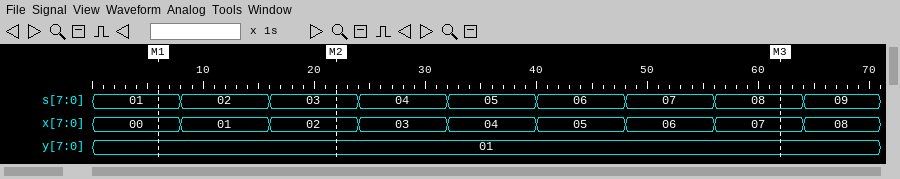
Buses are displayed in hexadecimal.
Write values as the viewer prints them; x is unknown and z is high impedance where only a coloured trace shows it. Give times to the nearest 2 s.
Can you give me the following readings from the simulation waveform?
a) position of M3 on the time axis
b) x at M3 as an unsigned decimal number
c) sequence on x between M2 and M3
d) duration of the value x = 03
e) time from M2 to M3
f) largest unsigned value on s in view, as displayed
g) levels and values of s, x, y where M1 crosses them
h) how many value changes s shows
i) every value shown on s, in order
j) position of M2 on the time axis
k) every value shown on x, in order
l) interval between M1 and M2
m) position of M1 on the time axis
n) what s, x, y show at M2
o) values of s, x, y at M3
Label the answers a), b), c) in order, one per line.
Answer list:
a) 62 s
b) 7
c) 02, 03, 04, 05, 06, 07
d) 8 s
e) 40 s
f) 09
g) s=01, x=00, y=01
h) 8
i) 01, 02, 03, 04, 05, 06, 07, 08, 09
j) 22 s
k) 00, 01, 02, 03, 04, 05, 06, 07, 08
l) 16 s
m) 6 s
n) s=03, x=02, y=01
o) s=08, x=07, y=01
